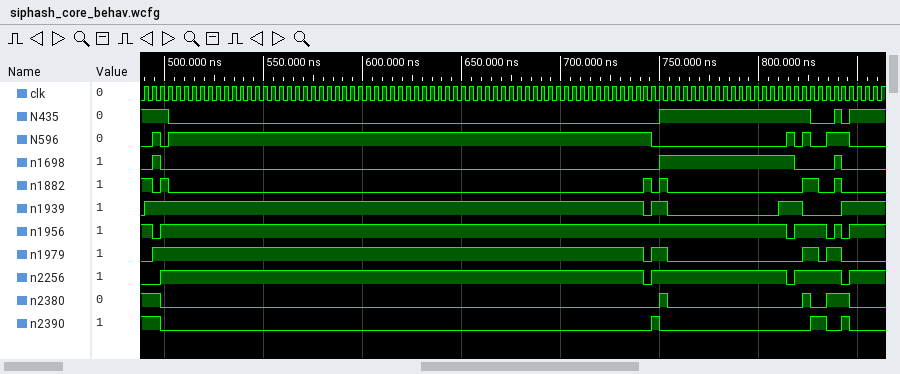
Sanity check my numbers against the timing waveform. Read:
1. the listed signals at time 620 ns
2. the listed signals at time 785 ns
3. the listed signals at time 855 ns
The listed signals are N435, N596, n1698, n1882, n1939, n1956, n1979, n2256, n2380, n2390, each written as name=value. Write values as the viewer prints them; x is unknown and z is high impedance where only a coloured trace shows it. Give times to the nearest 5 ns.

N435=0, N596=1, n1698=0, n1882=0, n1939=1, n1956=1, n1979=1, n2256=1, n2380=0, n2390=0
N435=1, N596=0, n1698=1, n1882=0, n1939=0, n1956=1, n1979=0, n2256=1, n2380=0, n2390=0
N435=1, N596=0, n1698=0, n1882=0, n1939=1, n1956=1, n1979=0, n2256=1, n2380=0, n2390=0
